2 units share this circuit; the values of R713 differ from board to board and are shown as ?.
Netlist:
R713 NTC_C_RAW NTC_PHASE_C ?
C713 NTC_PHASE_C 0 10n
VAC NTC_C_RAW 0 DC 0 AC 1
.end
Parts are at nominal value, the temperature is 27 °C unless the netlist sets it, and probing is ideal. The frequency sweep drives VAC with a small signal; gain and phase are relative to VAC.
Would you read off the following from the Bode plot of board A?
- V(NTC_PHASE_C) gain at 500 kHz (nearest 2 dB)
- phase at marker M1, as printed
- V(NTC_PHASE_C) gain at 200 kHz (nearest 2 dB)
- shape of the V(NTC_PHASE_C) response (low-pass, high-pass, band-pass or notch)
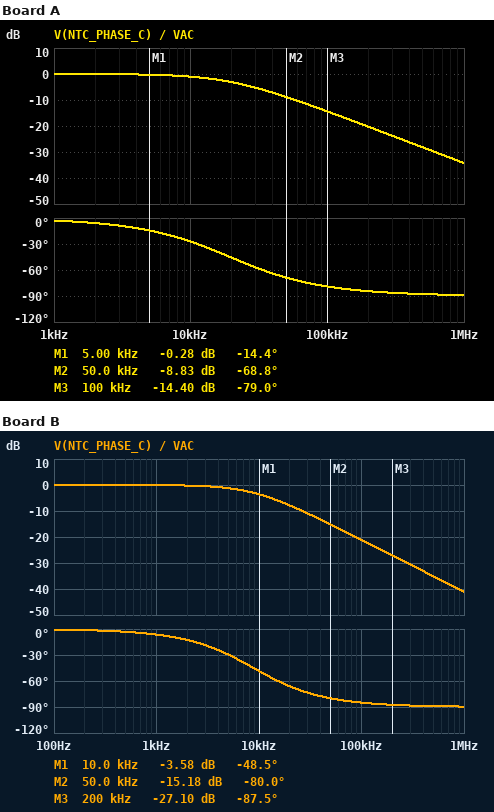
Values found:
-28 dB
-14.4 deg
-20 dB
low-pass
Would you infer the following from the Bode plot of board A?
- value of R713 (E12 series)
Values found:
820 Ω
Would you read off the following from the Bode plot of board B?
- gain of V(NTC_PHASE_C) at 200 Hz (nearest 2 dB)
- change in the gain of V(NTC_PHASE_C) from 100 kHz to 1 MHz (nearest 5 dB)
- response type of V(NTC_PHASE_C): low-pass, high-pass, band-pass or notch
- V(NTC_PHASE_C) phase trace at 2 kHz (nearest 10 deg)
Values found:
0 dB
-20 dB
low-pass
-10 deg
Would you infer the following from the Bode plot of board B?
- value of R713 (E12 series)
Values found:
1.8 kΩ
